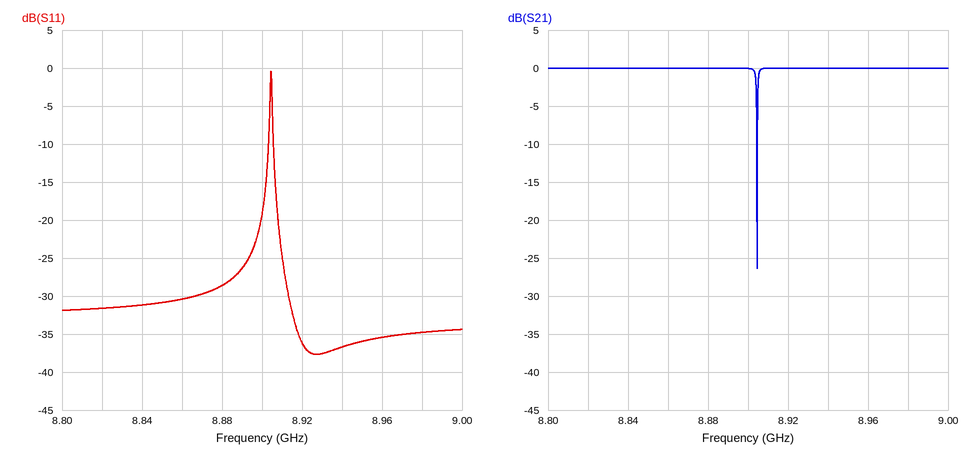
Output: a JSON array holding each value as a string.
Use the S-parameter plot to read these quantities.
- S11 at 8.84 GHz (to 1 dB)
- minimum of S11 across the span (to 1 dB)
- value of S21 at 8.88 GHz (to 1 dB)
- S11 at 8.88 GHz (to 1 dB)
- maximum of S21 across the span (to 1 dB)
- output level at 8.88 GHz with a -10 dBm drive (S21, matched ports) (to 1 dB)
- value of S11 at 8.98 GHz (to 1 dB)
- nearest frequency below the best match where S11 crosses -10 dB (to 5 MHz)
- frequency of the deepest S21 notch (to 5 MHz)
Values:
["-31 dB", "-38 dB", "0 dB", "-29 dB", "0 dB", "-10 dBm", "-35 dB", "8.905 GHz", "8.905 GHz"]
